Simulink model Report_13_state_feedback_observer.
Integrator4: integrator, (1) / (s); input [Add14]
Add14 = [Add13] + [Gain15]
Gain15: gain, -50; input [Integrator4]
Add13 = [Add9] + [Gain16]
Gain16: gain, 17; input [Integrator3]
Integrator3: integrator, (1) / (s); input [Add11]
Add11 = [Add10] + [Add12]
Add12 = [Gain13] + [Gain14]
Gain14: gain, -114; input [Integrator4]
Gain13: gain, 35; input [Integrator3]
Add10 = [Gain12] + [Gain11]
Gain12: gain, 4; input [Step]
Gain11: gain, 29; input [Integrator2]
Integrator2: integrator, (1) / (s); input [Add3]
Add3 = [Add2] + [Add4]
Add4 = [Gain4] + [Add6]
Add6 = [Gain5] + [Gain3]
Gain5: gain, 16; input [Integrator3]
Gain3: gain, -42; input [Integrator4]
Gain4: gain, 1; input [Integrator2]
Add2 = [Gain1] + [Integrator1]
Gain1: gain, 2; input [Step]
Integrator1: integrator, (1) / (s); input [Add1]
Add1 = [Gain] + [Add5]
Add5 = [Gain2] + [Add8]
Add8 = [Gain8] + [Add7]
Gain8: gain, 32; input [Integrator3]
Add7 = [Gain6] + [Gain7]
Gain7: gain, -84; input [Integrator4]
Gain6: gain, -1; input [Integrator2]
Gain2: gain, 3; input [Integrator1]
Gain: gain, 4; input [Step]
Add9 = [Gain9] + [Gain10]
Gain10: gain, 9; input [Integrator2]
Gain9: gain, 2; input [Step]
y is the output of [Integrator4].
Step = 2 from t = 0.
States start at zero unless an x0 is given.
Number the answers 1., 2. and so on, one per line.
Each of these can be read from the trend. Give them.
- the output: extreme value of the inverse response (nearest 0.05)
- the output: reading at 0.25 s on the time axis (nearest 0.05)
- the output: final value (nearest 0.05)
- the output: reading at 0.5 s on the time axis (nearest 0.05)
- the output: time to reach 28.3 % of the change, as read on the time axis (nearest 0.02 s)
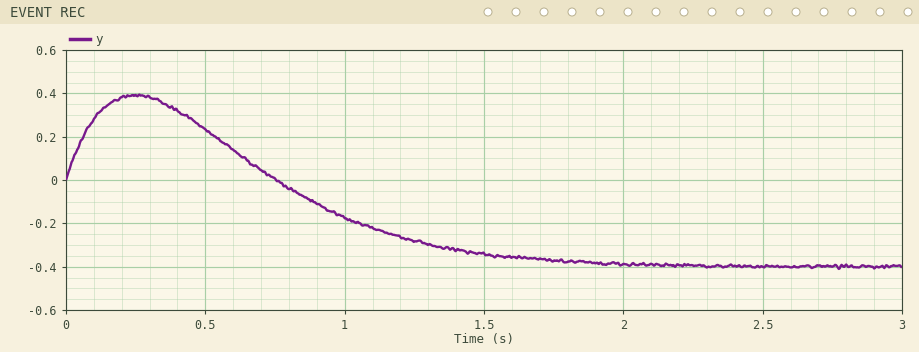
1. 0.40
2. 0.40
3. -0.40
4. 0.25
5. 0.90 s
